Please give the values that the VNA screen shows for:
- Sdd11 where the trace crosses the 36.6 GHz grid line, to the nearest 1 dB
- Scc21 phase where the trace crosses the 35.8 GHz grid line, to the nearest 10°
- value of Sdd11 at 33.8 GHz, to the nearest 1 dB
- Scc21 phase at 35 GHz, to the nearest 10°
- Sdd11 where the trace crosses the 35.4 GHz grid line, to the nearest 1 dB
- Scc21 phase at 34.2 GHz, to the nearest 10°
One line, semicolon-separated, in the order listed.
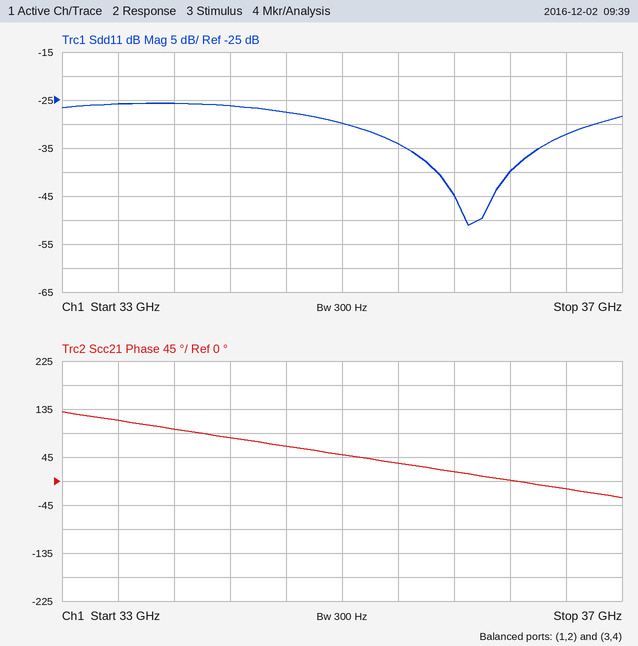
-32 dB; 20°; -26 dB; 50°; -34 dB; 80°
